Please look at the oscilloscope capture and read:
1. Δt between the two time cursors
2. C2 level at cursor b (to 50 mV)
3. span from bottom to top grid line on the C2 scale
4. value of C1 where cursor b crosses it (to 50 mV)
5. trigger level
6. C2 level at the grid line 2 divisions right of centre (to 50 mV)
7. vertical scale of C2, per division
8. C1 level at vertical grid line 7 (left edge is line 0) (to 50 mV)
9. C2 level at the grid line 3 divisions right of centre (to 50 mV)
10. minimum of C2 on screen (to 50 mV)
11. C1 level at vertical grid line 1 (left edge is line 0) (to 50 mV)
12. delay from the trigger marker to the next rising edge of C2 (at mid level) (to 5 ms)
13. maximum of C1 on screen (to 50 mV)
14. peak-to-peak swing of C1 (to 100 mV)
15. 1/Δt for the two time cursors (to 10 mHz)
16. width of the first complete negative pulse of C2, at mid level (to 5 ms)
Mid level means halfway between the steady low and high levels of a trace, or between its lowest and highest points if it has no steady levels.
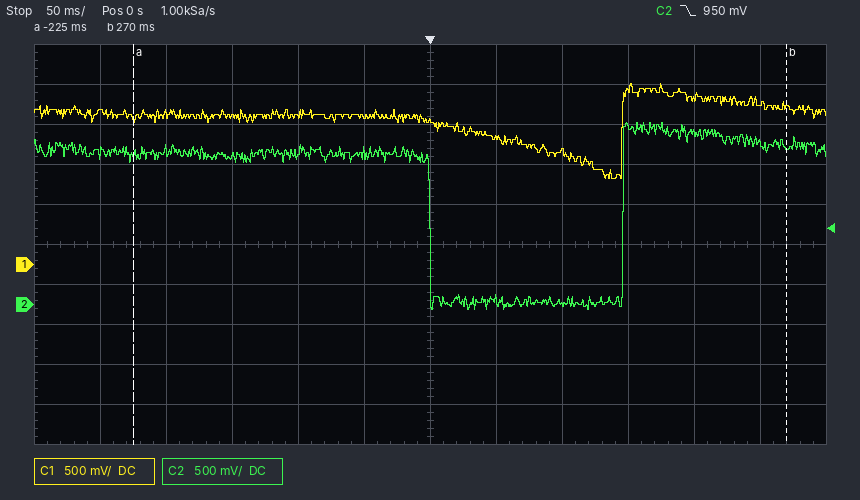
495 ms
1.95 V
5 V
2.00 V
950 mV
0 mV
500 mV
1.60 V
2.25 V
-50 mV
1.90 V
145 ms
2.25 V
1.20 V
2.02 Hz
145 ms
